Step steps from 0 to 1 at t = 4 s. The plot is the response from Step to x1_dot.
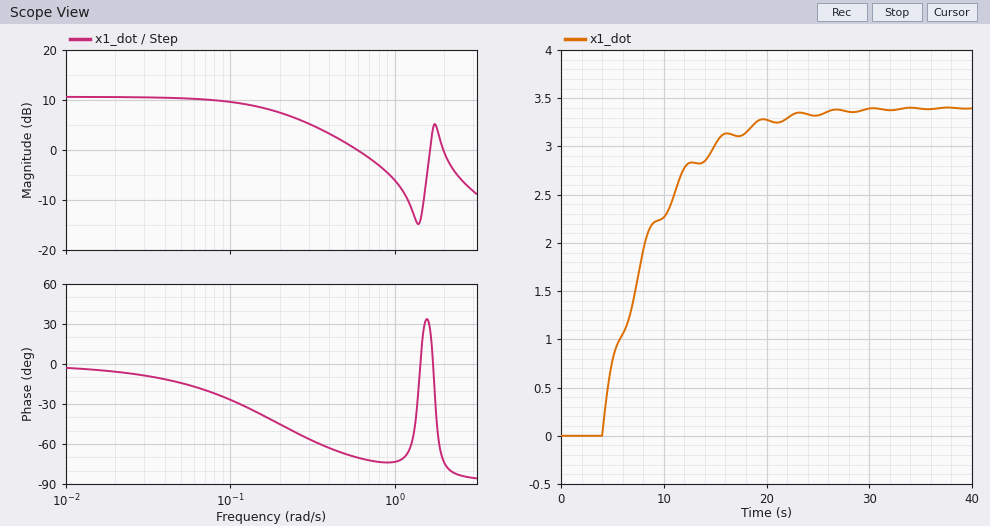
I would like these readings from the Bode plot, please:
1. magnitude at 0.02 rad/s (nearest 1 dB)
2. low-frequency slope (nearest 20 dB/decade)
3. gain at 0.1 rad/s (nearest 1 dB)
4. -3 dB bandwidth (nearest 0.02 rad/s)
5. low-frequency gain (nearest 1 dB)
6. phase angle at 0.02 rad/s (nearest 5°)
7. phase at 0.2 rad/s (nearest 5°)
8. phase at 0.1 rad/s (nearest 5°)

11 dB
0 dB/decade
10 dB
0.20 rad/s
11 dB
-5°
-45°
-25°
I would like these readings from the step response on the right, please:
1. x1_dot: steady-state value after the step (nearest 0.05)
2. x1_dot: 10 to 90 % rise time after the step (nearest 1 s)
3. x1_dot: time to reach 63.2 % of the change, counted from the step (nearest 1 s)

3.40
11 s
5 s
